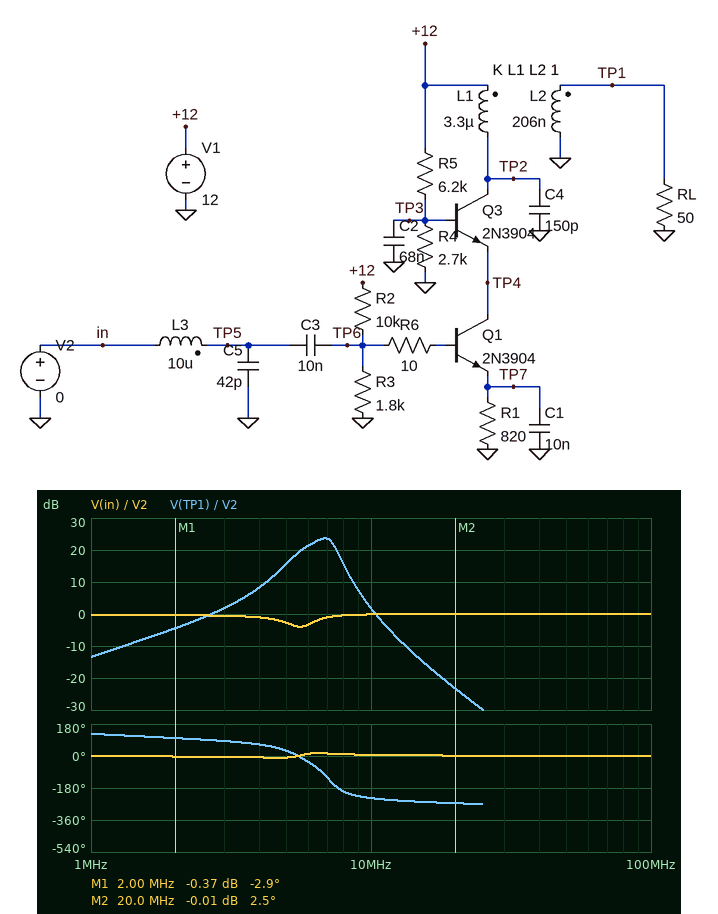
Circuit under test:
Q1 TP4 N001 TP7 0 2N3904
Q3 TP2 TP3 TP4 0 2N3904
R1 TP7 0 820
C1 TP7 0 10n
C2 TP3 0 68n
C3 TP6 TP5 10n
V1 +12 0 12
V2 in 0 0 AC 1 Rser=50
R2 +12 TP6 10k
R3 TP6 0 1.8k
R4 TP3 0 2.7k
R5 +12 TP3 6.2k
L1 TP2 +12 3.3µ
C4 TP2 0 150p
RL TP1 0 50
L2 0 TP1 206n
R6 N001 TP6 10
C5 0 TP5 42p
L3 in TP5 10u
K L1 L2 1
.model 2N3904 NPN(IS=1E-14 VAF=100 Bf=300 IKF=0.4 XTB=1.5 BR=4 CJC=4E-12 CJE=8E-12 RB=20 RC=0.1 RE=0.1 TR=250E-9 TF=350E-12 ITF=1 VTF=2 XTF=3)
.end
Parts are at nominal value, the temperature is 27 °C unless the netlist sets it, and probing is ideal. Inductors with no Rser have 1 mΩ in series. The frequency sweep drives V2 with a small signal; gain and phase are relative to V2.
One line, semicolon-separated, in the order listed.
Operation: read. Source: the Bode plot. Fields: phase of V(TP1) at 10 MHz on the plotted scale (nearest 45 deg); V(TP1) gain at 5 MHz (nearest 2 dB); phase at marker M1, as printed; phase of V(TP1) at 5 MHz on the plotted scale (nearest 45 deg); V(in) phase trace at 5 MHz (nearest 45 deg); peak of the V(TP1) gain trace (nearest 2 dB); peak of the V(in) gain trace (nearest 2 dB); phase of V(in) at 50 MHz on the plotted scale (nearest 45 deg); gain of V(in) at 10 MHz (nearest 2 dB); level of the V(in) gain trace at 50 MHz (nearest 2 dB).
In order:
-225 deg; 16 dB; -2.9 deg; 45 deg; 0 deg; 24 dB; 0 dB; 0 deg; 0 dB; 0 dB
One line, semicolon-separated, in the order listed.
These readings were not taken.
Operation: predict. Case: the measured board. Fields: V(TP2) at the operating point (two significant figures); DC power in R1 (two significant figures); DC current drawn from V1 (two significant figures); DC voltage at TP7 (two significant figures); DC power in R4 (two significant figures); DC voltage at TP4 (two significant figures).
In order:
12 V; 1.6 mW; 3.8 mA; 1.2 V; 4.9 mW; 3.0 V
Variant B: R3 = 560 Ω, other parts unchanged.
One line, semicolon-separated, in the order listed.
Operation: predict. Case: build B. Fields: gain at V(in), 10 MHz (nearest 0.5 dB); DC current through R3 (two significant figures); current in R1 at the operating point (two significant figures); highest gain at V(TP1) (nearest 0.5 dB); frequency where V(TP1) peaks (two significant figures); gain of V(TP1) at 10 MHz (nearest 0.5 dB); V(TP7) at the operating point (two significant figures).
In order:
-0.5 dB; 1.1 mA; 64 µA; -6.5 dB; 7.0 MHz; -24.0 dB; 53 mV
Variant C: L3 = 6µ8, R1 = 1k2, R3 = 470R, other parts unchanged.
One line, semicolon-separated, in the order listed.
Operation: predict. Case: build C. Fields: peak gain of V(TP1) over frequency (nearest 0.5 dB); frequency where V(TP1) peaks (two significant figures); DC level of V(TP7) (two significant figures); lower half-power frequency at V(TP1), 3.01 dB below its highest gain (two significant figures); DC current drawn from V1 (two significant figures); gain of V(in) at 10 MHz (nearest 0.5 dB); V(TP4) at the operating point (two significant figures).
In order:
-30.0 dB; 7.1 MHz; 9.5 mV; 6.4 MHz; 2.5 mA; -1.0 dB; 3.1 V
